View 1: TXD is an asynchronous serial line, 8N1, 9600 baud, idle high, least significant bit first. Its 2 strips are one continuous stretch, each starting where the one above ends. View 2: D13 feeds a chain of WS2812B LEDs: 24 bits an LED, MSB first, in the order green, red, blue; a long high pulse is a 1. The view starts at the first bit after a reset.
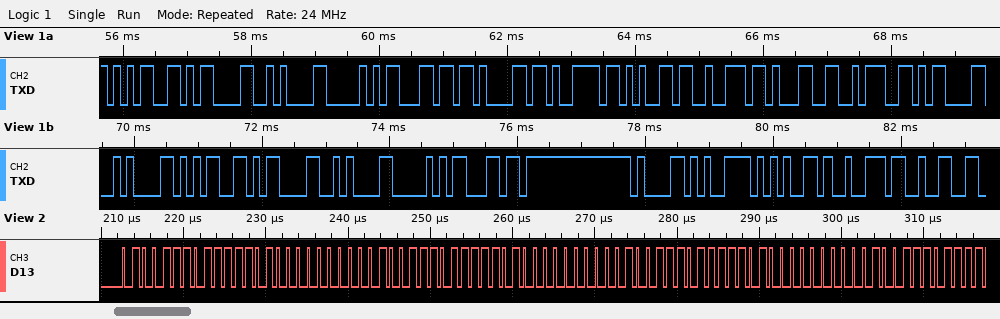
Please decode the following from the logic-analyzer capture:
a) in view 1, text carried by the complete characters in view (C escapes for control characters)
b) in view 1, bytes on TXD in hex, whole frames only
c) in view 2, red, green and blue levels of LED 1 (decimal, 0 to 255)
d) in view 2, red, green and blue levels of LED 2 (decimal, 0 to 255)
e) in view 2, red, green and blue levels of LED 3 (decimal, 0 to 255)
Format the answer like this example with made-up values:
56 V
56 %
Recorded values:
"5\r\nPlayer1:\r\n5\r\nPlayer2"
35 0D 0A 50 6C 61 79 65 72 31 3A 0D 0A 35 0D 0A 50 6C 61 79 65 72 32
250, 78, 0
250, 78, 0
250, 78, 0
